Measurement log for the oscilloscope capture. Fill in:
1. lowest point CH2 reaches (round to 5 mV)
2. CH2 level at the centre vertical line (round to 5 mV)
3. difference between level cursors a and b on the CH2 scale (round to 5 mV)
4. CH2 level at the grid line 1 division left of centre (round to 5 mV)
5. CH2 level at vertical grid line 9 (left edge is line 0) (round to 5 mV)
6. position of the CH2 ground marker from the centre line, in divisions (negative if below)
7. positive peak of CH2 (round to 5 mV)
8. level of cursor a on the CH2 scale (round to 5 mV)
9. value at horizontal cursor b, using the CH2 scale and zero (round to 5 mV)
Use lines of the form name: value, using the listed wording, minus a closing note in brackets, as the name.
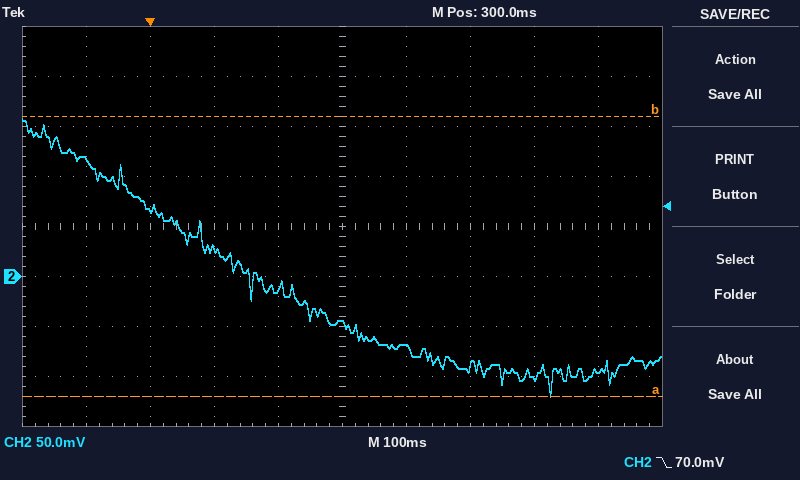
lowest point CH2 reaches: -120 mV
CH2 level at the centre vertical line: -45 mV
difference between level cursors a and b on the CH2 scale: 280 mV
CH2 level at the grid line 1 division left of centre: -10 mV
CH2 level at vertical grid line 9 (left edge is line 0): -95 mV
position of the CH2 ground marker from the centre line, in divisions: -1.0 div
positive peak of CH2: 160 mV
level of cursor a on the CH2 scale: -120 mV
value at horizontal cursor b, using the CH2 scale and zero: 160 mV
